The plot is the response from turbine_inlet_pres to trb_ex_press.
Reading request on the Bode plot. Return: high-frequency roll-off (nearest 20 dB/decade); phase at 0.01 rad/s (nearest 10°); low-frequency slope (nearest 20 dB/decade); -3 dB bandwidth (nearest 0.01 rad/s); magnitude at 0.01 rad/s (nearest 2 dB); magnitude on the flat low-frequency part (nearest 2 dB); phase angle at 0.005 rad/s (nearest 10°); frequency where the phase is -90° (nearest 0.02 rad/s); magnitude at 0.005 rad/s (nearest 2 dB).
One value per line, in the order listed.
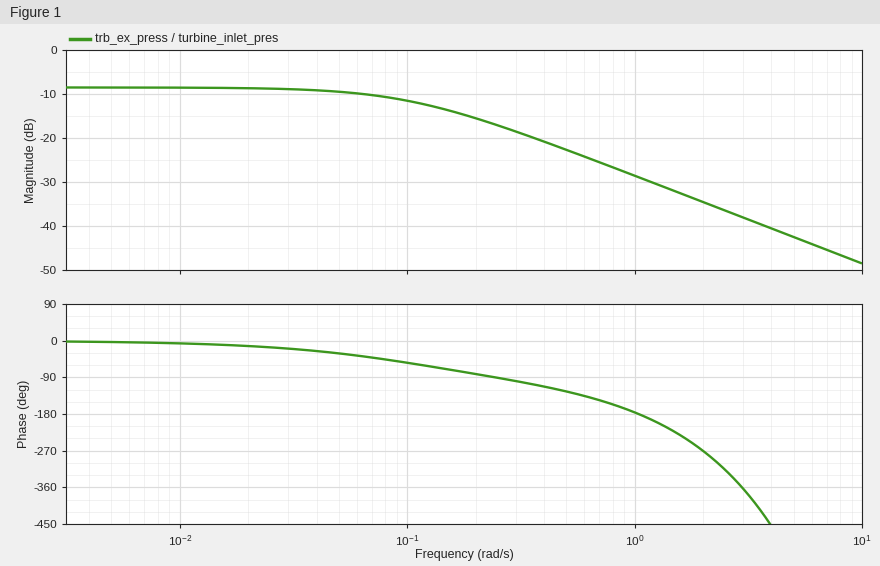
-20 dB/decade
-10°
0 dB/decade
0.10 rad/s
-8 dB
-8 dB
0°
0.24 rad/s
-8 dB
